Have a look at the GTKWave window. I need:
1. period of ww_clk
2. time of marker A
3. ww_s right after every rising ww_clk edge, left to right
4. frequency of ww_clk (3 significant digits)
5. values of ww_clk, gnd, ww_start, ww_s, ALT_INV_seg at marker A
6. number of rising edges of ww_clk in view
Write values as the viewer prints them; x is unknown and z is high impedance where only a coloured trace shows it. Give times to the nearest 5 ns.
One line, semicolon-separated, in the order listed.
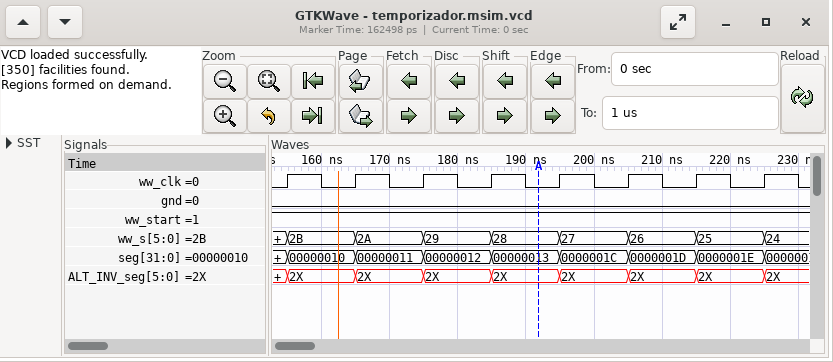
10 ns; 190 ns; 2B, 2A, 29, 28, 27, 26, 25, 24; 100 MHz; ww_clk=0, gnd=0, ww_start=1, ww_s=28, ALT_INV_seg=2X; 8
